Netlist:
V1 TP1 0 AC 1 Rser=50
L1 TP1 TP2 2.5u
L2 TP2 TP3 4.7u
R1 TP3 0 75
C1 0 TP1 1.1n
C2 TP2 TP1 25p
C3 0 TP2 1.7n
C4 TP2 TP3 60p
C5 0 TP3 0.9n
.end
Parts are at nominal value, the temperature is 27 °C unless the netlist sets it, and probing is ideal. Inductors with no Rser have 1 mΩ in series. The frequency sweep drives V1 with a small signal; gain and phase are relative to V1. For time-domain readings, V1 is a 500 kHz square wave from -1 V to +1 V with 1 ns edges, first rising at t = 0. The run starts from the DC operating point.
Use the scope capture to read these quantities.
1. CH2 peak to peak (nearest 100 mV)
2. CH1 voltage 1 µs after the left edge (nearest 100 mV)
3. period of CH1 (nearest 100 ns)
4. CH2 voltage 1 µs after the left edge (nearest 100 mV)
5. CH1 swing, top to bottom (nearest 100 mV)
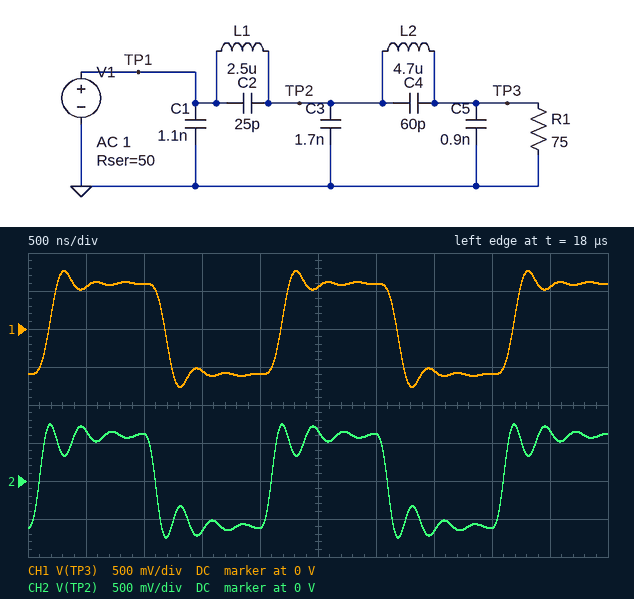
1.5 V
600 mV
2.0 µs
600 mV
1.5 V
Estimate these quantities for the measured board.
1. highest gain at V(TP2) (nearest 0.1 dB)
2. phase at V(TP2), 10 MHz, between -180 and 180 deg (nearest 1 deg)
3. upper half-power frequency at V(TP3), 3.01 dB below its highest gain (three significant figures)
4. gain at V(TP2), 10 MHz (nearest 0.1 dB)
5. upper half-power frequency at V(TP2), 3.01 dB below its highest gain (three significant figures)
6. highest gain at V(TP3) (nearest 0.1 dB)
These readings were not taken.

-0.3 dB
107 deg
3.62 MHz
-37.1 dB
4.11 MHz
-4.4 dB
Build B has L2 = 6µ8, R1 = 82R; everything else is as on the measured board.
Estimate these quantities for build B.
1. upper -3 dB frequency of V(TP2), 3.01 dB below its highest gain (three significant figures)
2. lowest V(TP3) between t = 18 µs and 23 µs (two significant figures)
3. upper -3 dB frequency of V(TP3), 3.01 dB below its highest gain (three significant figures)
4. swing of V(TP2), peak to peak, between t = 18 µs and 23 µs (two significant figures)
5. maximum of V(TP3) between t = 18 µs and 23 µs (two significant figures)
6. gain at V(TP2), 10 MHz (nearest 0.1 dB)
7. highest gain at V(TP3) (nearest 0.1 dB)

3.98 MHz
-750 mV
2.57 MHz
1.7 V
750 mV
-37.2 dB
-4.1 dB
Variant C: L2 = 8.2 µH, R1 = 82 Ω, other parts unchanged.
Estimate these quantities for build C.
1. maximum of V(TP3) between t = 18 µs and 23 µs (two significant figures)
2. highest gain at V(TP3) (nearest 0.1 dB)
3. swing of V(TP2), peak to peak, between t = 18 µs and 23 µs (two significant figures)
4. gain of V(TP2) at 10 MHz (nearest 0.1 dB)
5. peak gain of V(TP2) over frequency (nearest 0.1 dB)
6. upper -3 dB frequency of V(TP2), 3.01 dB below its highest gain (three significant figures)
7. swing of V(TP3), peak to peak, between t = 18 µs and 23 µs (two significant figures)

720 mV
-4.1 dB
1.8 V
-37.2 dB
-0.4 dB
3.94 MHz
1.4 V
